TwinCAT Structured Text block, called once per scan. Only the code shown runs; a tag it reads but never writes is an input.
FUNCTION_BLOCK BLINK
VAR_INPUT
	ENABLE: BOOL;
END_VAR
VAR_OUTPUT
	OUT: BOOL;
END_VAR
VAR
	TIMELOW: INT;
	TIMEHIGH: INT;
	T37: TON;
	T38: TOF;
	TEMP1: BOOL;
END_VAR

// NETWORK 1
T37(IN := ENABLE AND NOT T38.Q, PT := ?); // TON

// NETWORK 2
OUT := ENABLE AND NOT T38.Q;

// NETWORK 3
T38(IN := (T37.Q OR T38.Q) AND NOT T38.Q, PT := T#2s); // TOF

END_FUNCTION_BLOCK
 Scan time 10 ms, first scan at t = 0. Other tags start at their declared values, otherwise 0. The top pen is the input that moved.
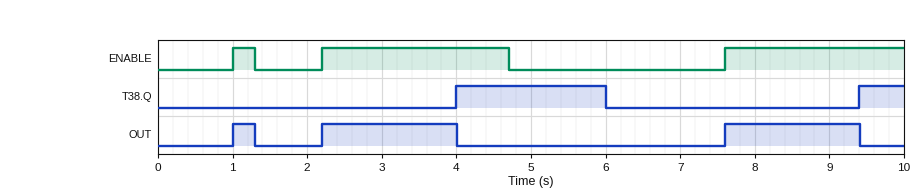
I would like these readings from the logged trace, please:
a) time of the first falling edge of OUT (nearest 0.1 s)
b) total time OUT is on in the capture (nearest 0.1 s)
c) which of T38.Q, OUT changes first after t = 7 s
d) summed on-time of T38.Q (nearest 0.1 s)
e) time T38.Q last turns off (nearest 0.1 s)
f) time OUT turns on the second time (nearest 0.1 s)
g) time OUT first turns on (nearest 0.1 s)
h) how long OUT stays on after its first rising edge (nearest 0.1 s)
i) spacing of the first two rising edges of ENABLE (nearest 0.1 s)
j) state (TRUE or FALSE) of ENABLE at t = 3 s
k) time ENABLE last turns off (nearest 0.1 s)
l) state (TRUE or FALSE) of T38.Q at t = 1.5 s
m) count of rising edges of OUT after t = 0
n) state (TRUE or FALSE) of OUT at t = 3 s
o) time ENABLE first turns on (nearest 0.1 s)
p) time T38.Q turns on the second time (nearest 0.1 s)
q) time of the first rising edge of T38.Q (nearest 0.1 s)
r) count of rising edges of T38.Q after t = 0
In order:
1.3 s
3.9 s
OUT
2.6 s
6.0 s
2.2 s
1.0 s
0.3 s
1.2 s
TRUE
4.7 s
FALSE
3
TRUE
1.0 s
9.4 s
4.0 s
2
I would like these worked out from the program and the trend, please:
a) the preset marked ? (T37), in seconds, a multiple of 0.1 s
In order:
1.8 s
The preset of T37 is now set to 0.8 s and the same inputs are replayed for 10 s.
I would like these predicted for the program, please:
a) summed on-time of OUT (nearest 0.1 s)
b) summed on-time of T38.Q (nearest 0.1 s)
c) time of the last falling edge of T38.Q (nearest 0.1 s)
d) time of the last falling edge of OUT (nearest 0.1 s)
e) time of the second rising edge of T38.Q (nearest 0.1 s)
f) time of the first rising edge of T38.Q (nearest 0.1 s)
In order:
1.9 s
3.6 s
5.0 s
8.4 s
8.4 s
3.0 s
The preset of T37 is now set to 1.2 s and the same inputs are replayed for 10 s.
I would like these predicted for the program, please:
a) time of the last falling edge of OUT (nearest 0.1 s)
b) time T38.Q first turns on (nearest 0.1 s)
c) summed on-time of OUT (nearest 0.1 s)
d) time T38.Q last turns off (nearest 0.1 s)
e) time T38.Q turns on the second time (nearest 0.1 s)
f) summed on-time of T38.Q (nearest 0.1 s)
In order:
8.8 s
3.4 s
2.7 s
5.4 s
8.8 s
3.2 s
